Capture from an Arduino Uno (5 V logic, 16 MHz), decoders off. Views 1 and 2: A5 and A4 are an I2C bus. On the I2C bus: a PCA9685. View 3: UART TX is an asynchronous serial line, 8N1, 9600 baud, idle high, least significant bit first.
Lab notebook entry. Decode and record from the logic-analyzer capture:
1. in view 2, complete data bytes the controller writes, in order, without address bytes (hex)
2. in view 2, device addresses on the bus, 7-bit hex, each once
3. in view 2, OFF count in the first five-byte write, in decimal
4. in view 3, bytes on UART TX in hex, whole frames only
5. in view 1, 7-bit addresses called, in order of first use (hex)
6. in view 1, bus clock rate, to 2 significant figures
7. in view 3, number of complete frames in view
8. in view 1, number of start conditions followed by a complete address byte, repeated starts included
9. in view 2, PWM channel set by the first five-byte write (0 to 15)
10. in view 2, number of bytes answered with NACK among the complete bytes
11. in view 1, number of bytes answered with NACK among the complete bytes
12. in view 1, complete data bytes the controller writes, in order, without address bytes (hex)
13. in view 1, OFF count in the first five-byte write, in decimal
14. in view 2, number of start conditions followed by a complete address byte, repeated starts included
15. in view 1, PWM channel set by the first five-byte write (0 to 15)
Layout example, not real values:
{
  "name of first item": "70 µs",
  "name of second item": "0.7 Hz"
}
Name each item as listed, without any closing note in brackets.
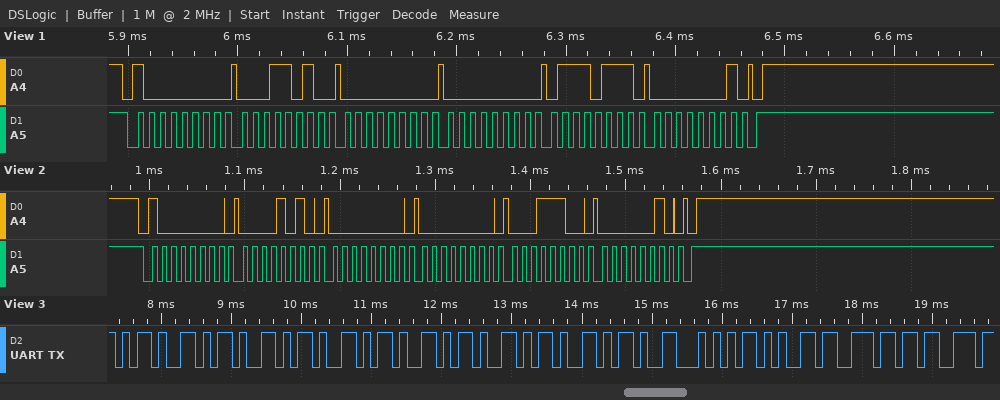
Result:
{
  "in view 2, complete data bytes the controller writes, in order, without address bytes": "0A 00 00 1C 02",
  "in view 2, device addresses on the bus, 7-bit hex, each once": "0x40",
  "in view 2, OFF count in the first five-byte write, in decimal": "540",
  "in view 3, bytes on UART TX in hex, whole frames only": "0x2D 0x2D 0x2D 0x2D 0x2D 0x2D 0x2D 0x54 0x65 0x6E 0x73",
  "in view 1, 7-bit addresses called, in order of first use": "0x40",
  "in view 1, bus clock rate, to 2 significant figures": "100 kHz",
  "in view 3, number of complete frames in view": "11",
  "in view 1, number of start conditions followed by a complete address byte, repeated starts included": "1",
  "in view 2, PWM channel set by the first five-byte write": "1",
  "in view 2, number of bytes answered with NACK among the complete bytes": "0",
  "in view 1, number of bytes answered with NACK among the complete bytes": "0",
  "in view 1, complete data bytes the controller writes, in order, without address bytes": "1A 00 00 77 01",
  "in view 1, OFF count in the first five-byte write, in decimal": "375",
  "in view 2, number of start conditions followed by a complete address byte, repeated starts included": "1",
  "in view 1, PWM channel set by the first five-byte write": "5"
}
